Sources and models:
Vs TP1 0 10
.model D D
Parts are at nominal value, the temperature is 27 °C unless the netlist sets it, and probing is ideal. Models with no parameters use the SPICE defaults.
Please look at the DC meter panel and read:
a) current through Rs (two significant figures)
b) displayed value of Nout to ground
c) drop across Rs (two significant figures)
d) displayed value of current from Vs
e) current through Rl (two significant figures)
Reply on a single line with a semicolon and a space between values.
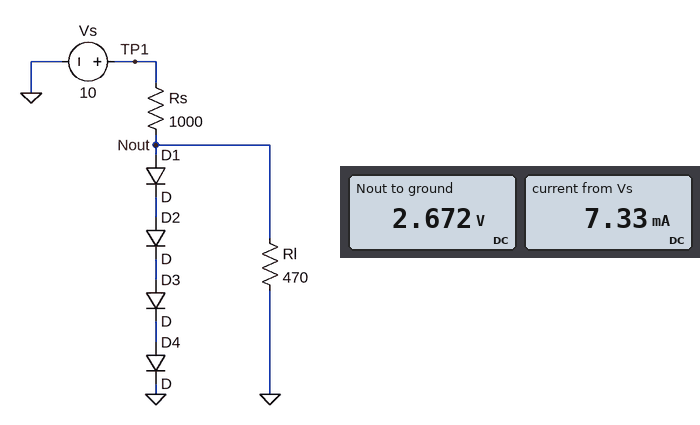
7.3 mA; 2.672 V; 7.3 V; 7.33 mA; 5.7 mA
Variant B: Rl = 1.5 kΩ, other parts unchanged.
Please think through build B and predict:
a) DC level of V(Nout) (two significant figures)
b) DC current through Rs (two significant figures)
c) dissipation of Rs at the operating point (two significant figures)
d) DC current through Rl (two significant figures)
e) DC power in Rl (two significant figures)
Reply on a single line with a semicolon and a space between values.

2.8 V; 7.2 mA; 52 mW; 1.9 mA; 5.2 mW
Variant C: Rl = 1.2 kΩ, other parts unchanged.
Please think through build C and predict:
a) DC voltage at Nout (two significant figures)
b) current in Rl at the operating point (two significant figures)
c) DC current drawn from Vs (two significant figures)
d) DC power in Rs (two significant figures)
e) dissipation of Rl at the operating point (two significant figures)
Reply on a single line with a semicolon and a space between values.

2.8 V; 2.3 mA; 7.2 mA; 52 mW; 6.5 mW
